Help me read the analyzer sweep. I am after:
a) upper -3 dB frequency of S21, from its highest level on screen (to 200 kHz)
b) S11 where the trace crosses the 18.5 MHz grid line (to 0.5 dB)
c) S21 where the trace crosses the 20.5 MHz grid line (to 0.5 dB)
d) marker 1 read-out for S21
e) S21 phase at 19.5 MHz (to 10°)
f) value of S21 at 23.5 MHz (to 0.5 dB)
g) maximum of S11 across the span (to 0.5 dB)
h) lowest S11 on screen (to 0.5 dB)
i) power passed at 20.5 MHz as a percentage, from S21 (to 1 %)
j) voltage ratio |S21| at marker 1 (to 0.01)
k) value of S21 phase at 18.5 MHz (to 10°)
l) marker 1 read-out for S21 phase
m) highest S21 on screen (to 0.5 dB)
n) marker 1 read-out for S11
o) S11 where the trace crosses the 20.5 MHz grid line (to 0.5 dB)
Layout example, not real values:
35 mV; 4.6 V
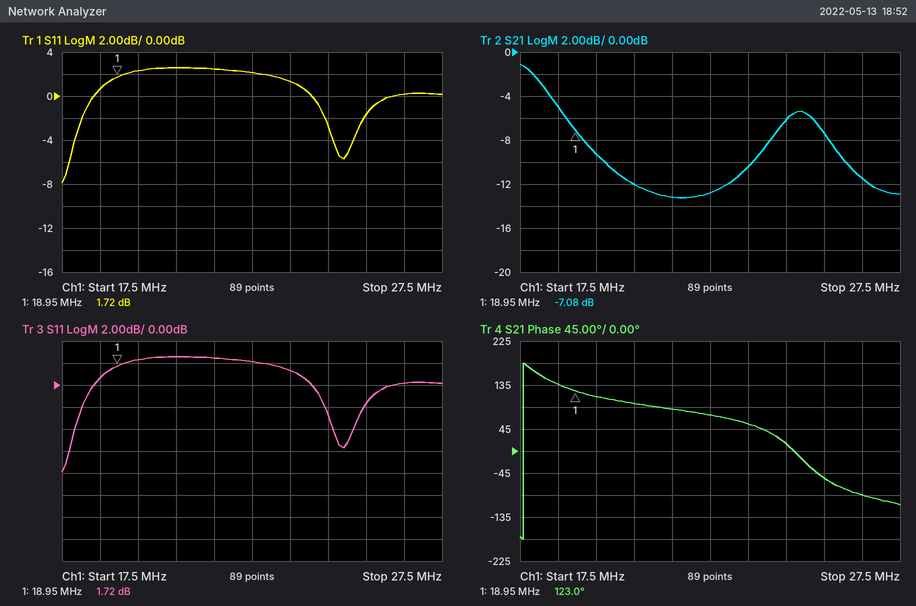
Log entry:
18.4 MHz; 0.5 dB; -12.0 dB; -7.08 dB; 110°; -10.5 dB; 2.5 dB; -8.0 dB; 6 %; 0.44; 140°; 123.0°; -1.0 dB; 1.72 dB; 2.5 dB
